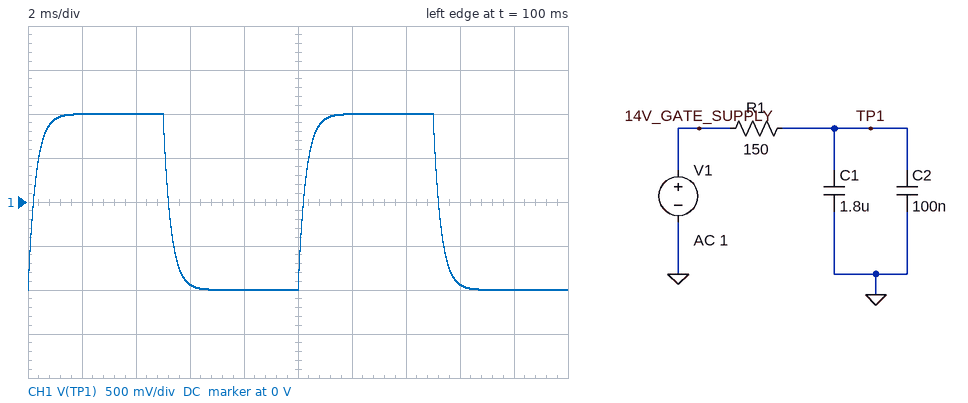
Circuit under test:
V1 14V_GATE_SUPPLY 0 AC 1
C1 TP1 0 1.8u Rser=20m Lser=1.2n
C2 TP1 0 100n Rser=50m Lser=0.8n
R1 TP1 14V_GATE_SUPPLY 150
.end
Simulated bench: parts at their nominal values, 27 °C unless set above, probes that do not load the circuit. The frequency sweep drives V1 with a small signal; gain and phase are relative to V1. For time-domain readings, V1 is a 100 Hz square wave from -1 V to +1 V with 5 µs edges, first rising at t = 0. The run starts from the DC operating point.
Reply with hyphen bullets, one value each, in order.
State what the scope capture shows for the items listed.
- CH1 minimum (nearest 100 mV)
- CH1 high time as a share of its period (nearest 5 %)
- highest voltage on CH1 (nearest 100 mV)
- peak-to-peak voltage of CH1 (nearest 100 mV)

- -1.0 V
- 50 %
- 1.0 V
- 2.0 V
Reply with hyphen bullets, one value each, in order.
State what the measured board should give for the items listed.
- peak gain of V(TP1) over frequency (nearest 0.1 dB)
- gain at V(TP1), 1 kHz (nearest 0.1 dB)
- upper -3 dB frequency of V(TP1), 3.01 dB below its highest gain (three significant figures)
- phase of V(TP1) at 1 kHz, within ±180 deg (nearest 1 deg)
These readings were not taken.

- 0 dB
- -6.2 dB
- 558 Hz
- -61 deg
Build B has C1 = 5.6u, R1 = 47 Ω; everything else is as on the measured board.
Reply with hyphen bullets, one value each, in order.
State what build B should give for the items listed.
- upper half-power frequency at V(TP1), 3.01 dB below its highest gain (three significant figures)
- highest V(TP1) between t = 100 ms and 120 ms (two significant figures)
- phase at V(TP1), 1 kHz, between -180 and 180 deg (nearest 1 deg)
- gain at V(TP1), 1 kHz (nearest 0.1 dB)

- 594 Hz
- 1.0 V
- -59 deg
- -5.8 dB
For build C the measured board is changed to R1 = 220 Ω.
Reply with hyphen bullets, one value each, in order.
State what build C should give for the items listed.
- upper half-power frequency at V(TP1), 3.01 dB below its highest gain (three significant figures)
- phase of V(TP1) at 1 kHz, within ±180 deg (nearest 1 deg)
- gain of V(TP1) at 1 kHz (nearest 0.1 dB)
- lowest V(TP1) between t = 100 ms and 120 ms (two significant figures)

- 381 Hz
- -69 deg
- -9.0 dB
- -1.0 V
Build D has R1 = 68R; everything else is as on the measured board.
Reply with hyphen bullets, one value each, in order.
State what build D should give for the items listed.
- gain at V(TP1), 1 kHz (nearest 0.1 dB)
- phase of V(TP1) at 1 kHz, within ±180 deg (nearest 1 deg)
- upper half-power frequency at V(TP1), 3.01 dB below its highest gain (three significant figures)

- -2.2 dB
- -39 deg
- 1.23 kHz
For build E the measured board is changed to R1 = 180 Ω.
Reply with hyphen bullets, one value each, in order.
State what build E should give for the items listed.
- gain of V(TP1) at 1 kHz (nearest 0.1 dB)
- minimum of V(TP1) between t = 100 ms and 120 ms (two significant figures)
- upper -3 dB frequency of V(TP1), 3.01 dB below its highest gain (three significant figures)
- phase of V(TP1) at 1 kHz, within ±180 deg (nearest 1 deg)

- -7.5 dB
- -1.0 V
- 465 Hz
- -65 deg
